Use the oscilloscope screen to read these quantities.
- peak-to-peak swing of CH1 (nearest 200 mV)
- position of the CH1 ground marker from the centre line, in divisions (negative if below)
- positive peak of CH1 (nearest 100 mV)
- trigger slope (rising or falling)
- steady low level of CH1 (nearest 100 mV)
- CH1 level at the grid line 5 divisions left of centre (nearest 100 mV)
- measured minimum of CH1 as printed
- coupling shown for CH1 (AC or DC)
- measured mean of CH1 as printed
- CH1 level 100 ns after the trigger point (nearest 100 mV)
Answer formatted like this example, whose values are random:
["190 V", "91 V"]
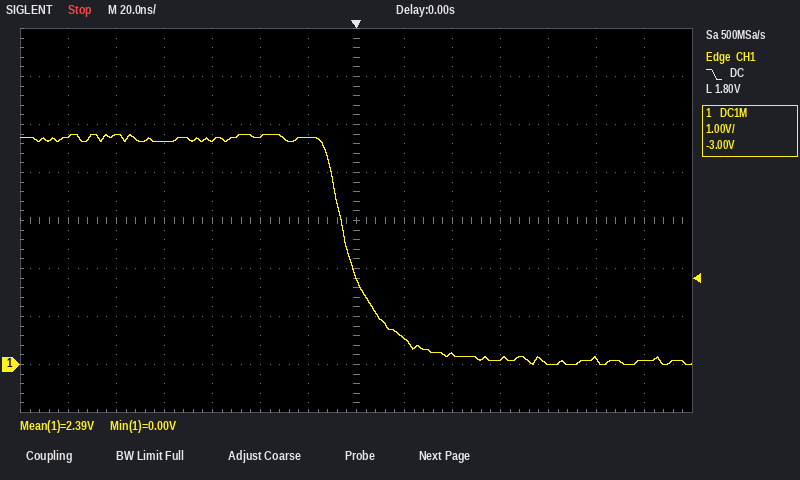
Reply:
["4.8 V", "-3.0 div", "4.8 V", "falling", "100 mV", "4.8 V", "0.00 V", "DC", "2.39 V", "100 mV"]
